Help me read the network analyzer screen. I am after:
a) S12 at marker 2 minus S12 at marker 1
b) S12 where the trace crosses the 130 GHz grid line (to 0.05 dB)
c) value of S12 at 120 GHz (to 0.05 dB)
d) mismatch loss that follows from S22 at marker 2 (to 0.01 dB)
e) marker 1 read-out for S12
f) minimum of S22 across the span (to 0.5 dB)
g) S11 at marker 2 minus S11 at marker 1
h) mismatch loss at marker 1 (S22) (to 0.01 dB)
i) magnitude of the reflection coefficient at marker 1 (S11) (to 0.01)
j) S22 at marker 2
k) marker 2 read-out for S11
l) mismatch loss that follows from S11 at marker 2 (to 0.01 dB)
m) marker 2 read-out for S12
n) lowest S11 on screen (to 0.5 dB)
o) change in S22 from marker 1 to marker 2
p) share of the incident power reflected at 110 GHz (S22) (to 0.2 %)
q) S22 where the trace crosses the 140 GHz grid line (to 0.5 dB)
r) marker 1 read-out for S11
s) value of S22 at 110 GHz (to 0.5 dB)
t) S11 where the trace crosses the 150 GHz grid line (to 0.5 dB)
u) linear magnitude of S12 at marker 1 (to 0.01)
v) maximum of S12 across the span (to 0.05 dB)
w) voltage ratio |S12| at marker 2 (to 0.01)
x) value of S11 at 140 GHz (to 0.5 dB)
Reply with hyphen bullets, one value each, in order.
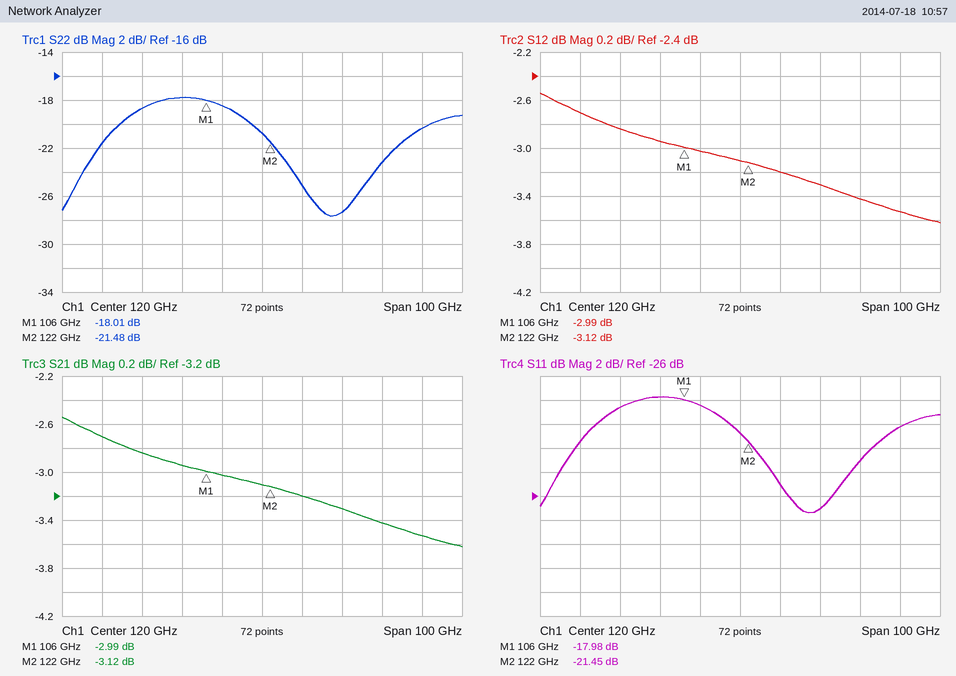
- -0.13 dB
- -3.20 dB
- -3.10 dB
- 0.03 dB
- -2.99 dB
- -27.5 dB
- -3.47 dB
- 0.07 dB
- 0.13
- -21.48 dB
- -21.45 dB
- 0.03 dB
- -3.12 dB
- -27.5 dB
- -3.47 dB
- 1.4 %
- -27.5 dB
- -17.98 dB
- -18.5 dB
- -23.0 dB
- 0.71
- -2.55 dB
- 0.70
- -27.0 dB
